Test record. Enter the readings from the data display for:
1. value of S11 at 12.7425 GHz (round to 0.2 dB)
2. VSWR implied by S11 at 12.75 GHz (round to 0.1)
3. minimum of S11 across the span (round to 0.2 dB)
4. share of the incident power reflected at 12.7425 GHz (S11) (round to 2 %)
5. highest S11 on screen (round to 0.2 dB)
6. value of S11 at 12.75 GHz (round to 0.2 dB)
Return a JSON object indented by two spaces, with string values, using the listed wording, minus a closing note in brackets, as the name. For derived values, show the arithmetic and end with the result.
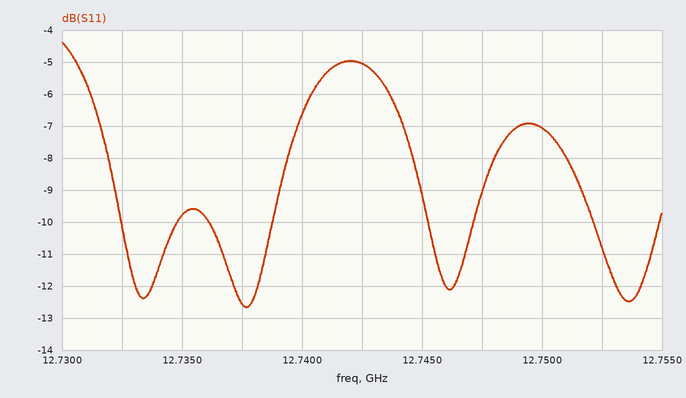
{
  "value of S11 at 12.7425 GHz": "-5.0 dB",
  "VSWR implied by S11 at 12.75 GHz": "|Γ| = 10^(-7/20) = 0.4467; VSWR = (1 + 0.4467)/(1 − 0.4467) ≈ 2.6",
  "minimum of S11 across the span": "-12.6 dB",
  "share of the incident power reflected at 12.7425 GHz (S11)": "10^(-5/10) ≈ 32 %",
  "highest S11 on screen": "-4.4 dB",
  "value of S11 at 12.75 GHz": "-7.0 dB"
}
